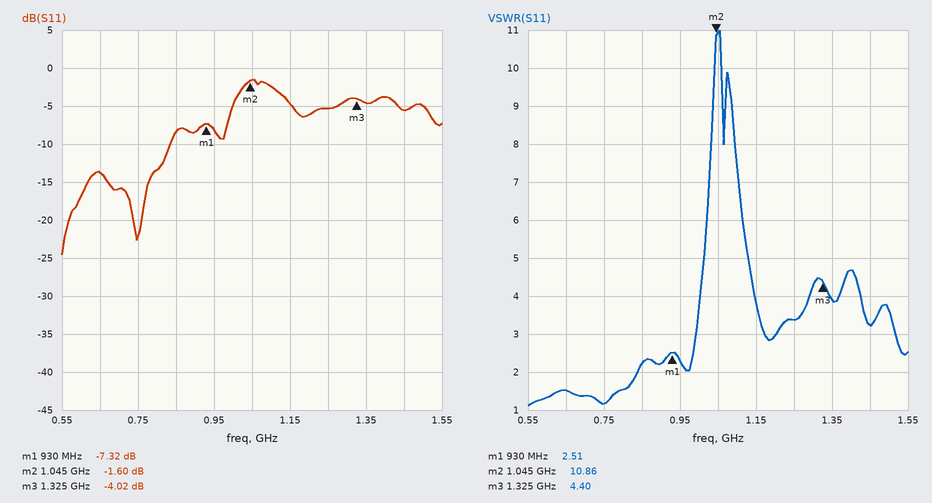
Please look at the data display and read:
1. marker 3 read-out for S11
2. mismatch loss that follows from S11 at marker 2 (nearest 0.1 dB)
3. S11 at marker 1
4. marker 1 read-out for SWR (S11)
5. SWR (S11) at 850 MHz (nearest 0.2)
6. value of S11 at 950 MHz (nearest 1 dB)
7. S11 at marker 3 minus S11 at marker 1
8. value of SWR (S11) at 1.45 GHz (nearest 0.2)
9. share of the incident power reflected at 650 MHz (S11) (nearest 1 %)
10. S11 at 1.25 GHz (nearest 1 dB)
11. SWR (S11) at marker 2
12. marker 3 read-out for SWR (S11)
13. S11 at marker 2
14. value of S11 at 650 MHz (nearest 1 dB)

-4.02 dB
5.1 dB
-7.32 dB
2.51
2.2
-8 dB
3.30 dB
3.2
4 %
-5 dB
10.86
4.40
-1.60 dB
-14 dB
